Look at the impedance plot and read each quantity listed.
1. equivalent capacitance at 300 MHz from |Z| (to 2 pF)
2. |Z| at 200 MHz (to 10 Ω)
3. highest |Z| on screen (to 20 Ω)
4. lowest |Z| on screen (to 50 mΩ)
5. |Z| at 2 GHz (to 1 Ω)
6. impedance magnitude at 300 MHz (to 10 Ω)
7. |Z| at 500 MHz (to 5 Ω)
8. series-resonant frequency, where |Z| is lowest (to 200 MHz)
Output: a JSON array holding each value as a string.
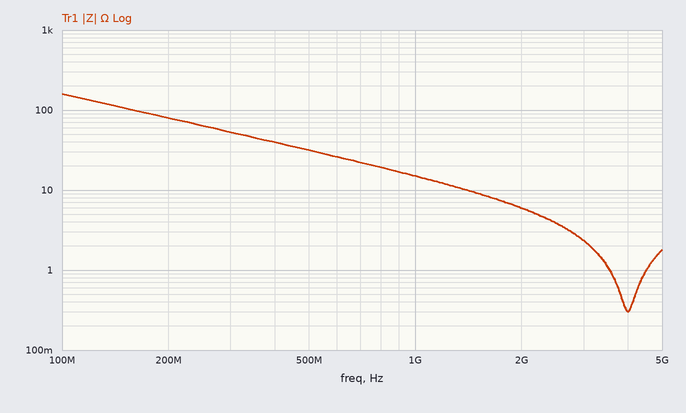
["10 pF", "80 Ω", "160 Ω", "300 mΩ", "6 Ω", "50 Ω", "30 Ω", "4.0 GHz"]
